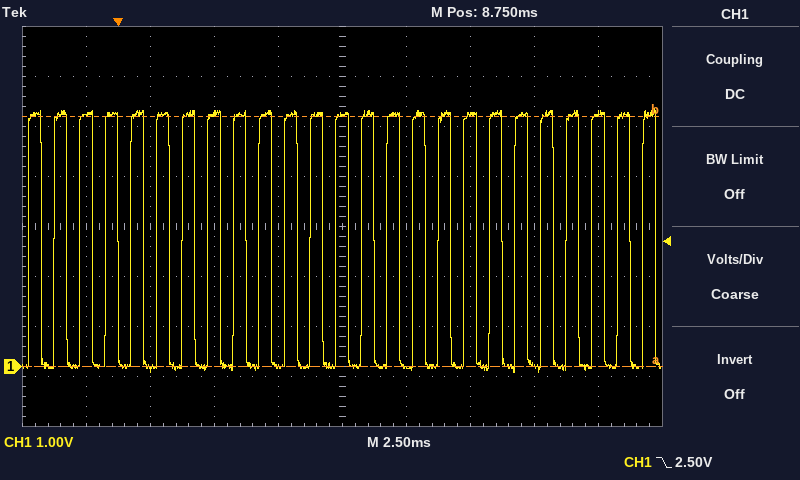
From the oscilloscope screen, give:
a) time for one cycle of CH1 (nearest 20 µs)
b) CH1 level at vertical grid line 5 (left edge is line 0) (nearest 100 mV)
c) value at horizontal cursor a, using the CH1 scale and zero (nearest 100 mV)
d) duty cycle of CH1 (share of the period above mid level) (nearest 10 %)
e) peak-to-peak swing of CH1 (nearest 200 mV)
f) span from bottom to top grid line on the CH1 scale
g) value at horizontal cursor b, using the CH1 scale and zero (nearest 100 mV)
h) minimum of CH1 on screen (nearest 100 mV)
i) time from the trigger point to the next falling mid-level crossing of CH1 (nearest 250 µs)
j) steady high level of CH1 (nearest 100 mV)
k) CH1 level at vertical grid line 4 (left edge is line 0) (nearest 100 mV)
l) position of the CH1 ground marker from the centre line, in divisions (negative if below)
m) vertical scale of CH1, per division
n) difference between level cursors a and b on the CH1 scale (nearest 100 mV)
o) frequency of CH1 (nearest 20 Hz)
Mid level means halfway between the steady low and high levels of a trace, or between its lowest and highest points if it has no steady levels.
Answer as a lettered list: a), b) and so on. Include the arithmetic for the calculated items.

a) 1.00 ms
b) 5.0 V
c) 0.0 V
d) 50 %
e) 5.2 V
f) 8 V
g) 5.0 V
h) -100 mV
i) 1.00 ms
j) 5.0 V
k) 0.0 V
l) -2.8 div
m) 1 V
n) 5.0 V
o) 1 / 1.00 ms ≈ 1.00 kHz
